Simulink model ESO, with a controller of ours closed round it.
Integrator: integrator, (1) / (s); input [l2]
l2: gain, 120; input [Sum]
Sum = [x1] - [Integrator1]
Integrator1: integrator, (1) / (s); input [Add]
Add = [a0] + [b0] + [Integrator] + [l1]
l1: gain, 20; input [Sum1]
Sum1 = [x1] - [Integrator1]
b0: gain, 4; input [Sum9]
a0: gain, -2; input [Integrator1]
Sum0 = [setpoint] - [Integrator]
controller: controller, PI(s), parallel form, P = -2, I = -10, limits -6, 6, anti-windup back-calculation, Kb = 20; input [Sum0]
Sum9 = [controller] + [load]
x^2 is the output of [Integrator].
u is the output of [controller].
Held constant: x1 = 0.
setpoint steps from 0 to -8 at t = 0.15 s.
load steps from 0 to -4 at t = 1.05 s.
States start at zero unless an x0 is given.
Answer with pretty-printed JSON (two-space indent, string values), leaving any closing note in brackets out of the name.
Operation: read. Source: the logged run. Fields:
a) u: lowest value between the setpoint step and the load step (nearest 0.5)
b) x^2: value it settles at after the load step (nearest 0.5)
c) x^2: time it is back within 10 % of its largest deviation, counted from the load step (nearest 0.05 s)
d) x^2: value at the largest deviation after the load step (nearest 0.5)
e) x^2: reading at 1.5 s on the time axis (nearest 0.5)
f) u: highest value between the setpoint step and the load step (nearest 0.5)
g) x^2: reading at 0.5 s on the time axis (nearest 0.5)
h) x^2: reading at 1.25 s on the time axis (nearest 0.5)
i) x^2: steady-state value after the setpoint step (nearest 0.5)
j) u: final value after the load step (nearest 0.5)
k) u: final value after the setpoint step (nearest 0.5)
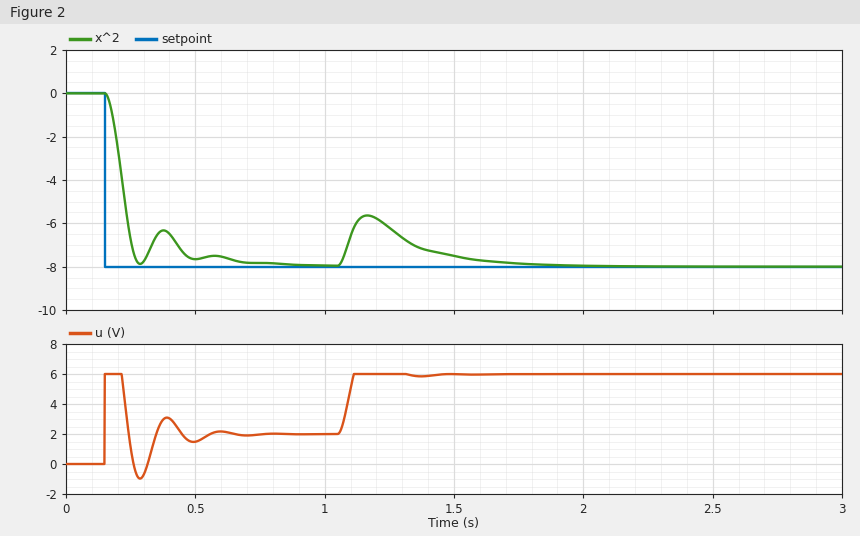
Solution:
{
  "u: lowest value between the setpoint step and the load step": "-1.0",
  "x^2: value it settles at after the load step": "-8.0",
  "x^2: time it is back within 10 % of its largest deviation, counted from the load step": "0.60 s",
  "x^2: value at the largest deviation after the load step": "-5.5",
  "x^2: reading at 1.5 s on the time axis": "-7.5",
  "u: highest value between the setpoint step and the load step": "6.0",
  "x^2: reading at 0.5 s on the time axis": "-7.5",
  "x^2: reading at 1.25 s on the time axis": "-6.0",
  "x^2: steady-state value after the setpoint step": "-8.0",
  "u: final value after the load step": "6.0",
  "u: final value after the setpoint step": "2.0"
}
